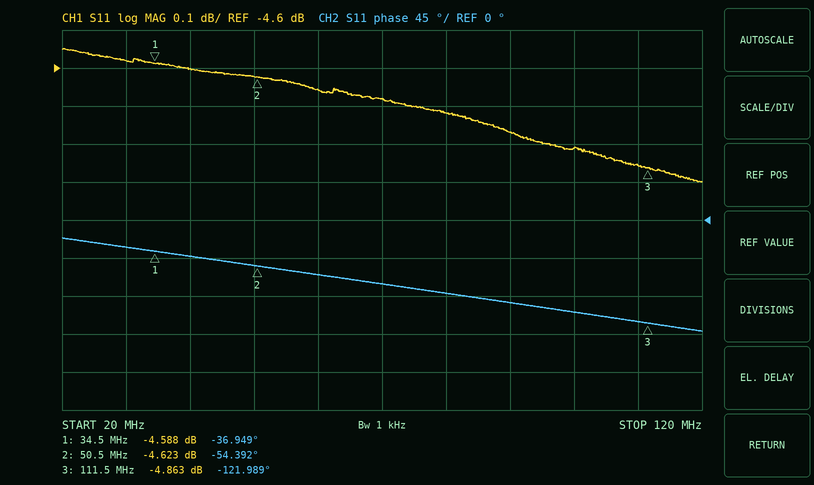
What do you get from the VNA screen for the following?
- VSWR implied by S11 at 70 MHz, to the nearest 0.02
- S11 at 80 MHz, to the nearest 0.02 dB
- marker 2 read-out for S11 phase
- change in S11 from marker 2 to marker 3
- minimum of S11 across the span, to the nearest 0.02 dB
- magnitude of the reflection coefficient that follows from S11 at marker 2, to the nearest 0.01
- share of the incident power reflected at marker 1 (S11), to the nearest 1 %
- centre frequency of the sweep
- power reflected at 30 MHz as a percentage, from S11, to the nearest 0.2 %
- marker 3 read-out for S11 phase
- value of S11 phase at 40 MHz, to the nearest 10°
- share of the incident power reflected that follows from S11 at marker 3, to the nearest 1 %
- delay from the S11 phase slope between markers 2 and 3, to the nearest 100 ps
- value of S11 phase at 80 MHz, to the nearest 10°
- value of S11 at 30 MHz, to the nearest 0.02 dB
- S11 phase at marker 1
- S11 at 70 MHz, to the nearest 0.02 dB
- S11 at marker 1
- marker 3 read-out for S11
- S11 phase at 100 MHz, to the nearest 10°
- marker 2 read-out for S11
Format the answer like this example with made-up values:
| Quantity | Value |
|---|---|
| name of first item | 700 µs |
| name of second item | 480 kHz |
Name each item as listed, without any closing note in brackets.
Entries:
| Quantity | Value |
|---|---|
| VSWR implied by S11 at 70 MHz, to the nearest 0.02 | 3.80 |
| S11 at 80 MHz, to the nearest 0.02 dB | -4.72 dB |
| marker 2 read-out for S11 phase | -54.392° |
| change in S11 from marker 2 to marker 3 | -0.240 dB |
| minimum of S11 across the span, to the nearest 0.02 dB | -4.90 dB |
| magnitude of the reflection coefficient that follows from S11 at marker 2, to the nearest 0.01 | 0.59 |
| share of the incident power reflected at marker 1 (S11), to the nearest 1 % | 35 % |
| centre frequency of the sweep | 70 MHz |
| power reflected at 30 MHz as a percentage, from S11, to the nearest 0.2 % | 34.8 % |
| marker 3 read-out for S11 phase | -121.989° |
| value of S11 phase at 40 MHz, to the nearest 10° | -40° |
| share of the incident power reflected that follows from S11 at marker 3, to the nearest 1 % | 33 % |
| delay from the S11 phase slope between markers 2 and 3, to the nearest 100 ps | 3.1 ns |
| value of S11 phase at 80 MHz, to the nearest 10° | -90° |
| value of S11 at 30 MHz, to the nearest 0.02 dB | -4.58 dB |
| S11 phase at marker 1 | -36.949° |
| S11 at 70 MHz, to the nearest 0.02 dB | -4.68 dB |
| S11 at marker 1 | -4.588 dB |
| marker 3 read-out for S11 | -4.863 dB |
| S11 phase at 100 MHz, to the nearest 10° | -110° |
| marker 2 read-out for S11 | -4.623 dB |
